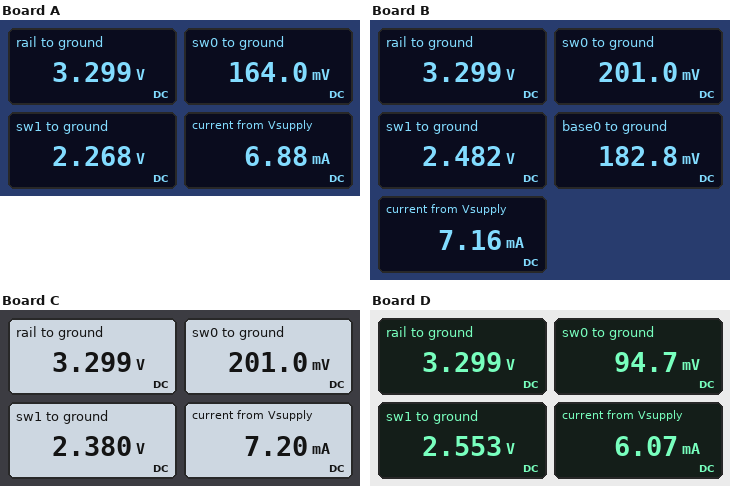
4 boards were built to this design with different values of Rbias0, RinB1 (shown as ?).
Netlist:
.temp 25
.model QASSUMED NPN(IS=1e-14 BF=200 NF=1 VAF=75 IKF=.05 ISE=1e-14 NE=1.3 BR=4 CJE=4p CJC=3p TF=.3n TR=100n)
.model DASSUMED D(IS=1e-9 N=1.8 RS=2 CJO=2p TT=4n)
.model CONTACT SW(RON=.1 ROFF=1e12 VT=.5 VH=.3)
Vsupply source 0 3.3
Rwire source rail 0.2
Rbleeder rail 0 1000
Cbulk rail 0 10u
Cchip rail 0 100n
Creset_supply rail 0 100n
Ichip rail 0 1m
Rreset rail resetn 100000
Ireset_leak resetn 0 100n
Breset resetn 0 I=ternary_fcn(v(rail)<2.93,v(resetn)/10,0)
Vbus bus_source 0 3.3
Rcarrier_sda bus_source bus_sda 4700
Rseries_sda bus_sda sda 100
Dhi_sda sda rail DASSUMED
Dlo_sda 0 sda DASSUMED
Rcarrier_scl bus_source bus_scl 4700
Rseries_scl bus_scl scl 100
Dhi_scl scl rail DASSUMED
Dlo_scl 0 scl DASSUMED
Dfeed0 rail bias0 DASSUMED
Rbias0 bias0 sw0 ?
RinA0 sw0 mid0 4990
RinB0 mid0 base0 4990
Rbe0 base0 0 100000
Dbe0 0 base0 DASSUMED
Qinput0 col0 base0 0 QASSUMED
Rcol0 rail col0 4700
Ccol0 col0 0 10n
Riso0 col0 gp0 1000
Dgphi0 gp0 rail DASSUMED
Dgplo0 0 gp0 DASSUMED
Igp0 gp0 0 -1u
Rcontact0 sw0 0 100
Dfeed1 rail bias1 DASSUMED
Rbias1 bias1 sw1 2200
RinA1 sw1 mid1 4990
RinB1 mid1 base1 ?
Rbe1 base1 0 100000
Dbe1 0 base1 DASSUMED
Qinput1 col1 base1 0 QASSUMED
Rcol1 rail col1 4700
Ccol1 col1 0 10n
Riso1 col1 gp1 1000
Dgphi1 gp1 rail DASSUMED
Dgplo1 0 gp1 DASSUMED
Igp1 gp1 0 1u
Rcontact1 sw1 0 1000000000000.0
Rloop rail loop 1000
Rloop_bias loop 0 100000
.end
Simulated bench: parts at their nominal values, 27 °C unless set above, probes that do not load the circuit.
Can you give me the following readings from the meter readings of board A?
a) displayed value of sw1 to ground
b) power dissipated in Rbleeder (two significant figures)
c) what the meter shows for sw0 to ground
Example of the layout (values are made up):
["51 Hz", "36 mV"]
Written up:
["2.268 V", "11 mW", "164.0 mV"]
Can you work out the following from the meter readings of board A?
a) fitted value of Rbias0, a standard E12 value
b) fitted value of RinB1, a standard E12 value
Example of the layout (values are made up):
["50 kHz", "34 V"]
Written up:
["1.5 kΩ", "2.7 kΩ"]
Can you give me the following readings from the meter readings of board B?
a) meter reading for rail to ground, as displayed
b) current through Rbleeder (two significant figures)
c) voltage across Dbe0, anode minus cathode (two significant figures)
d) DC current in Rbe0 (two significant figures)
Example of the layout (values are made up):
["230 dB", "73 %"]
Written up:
["3.299 V", "3.3 mA", "-180 mV", "1.8 µA"]
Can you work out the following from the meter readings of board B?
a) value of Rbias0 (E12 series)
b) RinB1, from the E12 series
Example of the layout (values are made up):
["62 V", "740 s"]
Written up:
["1.2 kΩ", "10 kΩ"]
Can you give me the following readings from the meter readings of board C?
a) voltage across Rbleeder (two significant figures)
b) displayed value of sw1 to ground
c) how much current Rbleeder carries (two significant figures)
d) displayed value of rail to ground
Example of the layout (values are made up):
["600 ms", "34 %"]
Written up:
["3.3 V", "2.380 V", "3.3 mA", "3.299 V"]
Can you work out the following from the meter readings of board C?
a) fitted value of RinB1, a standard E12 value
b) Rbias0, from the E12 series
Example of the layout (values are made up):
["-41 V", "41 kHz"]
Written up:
["5.6 kΩ", "1.2 kΩ"]
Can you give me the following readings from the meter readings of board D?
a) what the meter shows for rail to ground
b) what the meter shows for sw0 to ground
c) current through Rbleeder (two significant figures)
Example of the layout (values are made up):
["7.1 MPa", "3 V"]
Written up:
["3.299 V", "94.7 mV", "3.3 mA"]
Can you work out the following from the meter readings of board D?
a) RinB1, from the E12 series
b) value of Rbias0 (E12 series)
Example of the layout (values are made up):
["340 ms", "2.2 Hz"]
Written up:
["15 kΩ", "2.7 kΩ"]
